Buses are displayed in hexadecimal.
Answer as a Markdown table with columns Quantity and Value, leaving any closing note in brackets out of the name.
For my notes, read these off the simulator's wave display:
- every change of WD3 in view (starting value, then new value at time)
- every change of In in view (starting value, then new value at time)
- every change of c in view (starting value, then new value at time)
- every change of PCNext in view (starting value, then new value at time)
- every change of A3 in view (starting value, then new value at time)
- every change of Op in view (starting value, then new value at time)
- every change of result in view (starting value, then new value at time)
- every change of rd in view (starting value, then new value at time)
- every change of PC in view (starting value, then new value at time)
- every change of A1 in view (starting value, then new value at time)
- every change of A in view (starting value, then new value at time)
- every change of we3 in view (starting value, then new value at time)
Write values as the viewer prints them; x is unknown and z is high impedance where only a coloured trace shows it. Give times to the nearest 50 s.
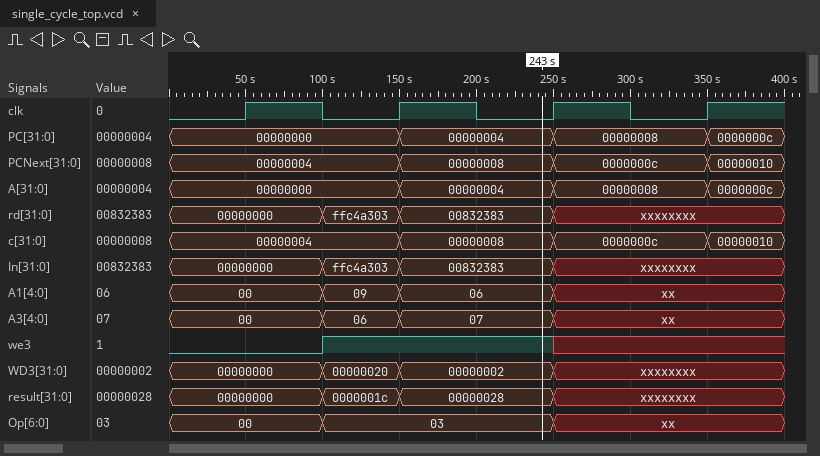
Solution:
| Quantity | Value |
|---|---|
| every change of WD3 in view | 00000000, 00000020 at 100 s, 00000002 at 150 s, xxxxxxxx at 250 s |
| every change of In in view | 00000000, ffc4a303 at 100 s, 00832383 at 150 s, xxxxxxxx at 250 s |
| every change of c in view | 00000004, 00000008 at 150 s, 0000000c at 250 s, 00000010 at 350 s |
| every change of PCNext in view | 00000004, 00000008 at 150 s, 0000000c at 250 s, 00000010 at 350 s |
| every change of A3 in view | 00, 06 at 100 s, 07 at 150 s, xx at 250 s |
| every change of Op in view | 00, 03 at 100 s, xx at 250 s |
| every change of result in view | 00000000, 0000001c at 100 s, 00000028 at 150 s, xxxxxxxx at 250 s |
| every change of rd in view | 00000000, ffc4a303 at 100 s, 00832383 at 150 s, xxxxxxxx at 250 s |
| every change of PC in view | 00000000, 00000004 at 150 s, 00000008 at 250 s, 0000000c at 350 s |
| every change of A1 in view | 00, 09 at 100 s, 06 at 150 s, xx at 250 s |
| every change of A in view | 00000000, 00000004 at 150 s, 00000008 at 250 s, 0000000c at 350 s |
| every change of we3 in view | 0, 1 at 100 s, x at 250 s |
